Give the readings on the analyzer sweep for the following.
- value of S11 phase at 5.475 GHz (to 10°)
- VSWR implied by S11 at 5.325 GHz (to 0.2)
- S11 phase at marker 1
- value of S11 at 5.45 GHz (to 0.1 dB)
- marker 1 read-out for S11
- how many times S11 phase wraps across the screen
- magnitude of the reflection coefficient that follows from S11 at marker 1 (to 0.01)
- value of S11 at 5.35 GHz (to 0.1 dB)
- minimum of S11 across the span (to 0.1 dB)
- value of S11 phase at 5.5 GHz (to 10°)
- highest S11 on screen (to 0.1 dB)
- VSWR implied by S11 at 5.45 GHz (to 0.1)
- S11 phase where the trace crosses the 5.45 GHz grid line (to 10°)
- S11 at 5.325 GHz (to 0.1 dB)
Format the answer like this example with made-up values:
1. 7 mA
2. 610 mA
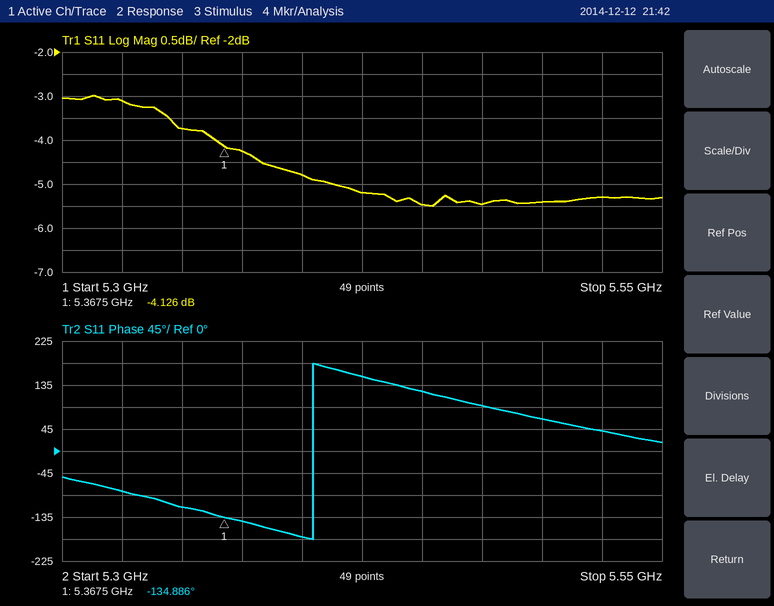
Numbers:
1. 90°
2. 5.6
3. -134.886°
4. -5.5 dB
5. -4.126 dB
6. 1
7. 0.62
8. -3.7 dB
9. -5.5 dB
10. 70°
11. -3.0 dB
12. 3.3
13. 120°
14. -3.1 dB
